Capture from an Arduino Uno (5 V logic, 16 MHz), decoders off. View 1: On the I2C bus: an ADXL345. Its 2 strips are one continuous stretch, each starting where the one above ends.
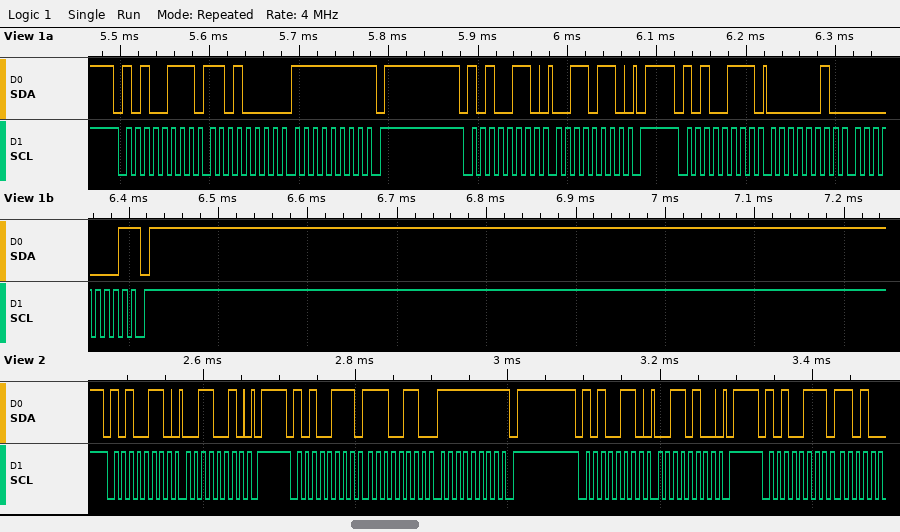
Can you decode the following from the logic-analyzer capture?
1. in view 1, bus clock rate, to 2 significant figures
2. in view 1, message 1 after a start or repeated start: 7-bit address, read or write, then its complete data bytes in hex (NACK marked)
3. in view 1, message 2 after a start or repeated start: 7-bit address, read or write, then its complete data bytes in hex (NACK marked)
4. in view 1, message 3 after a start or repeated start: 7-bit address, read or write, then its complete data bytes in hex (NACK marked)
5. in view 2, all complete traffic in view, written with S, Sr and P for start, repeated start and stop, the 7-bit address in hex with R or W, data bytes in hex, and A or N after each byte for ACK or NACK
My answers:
100 kHz
0x53 read: D0 FF NACK
0x53 write: 36
0x53 read: 02 01 NACK
S 53W A 32 A P S 53R A E6 A FF N P S 53W A 34 A P S 53R A
